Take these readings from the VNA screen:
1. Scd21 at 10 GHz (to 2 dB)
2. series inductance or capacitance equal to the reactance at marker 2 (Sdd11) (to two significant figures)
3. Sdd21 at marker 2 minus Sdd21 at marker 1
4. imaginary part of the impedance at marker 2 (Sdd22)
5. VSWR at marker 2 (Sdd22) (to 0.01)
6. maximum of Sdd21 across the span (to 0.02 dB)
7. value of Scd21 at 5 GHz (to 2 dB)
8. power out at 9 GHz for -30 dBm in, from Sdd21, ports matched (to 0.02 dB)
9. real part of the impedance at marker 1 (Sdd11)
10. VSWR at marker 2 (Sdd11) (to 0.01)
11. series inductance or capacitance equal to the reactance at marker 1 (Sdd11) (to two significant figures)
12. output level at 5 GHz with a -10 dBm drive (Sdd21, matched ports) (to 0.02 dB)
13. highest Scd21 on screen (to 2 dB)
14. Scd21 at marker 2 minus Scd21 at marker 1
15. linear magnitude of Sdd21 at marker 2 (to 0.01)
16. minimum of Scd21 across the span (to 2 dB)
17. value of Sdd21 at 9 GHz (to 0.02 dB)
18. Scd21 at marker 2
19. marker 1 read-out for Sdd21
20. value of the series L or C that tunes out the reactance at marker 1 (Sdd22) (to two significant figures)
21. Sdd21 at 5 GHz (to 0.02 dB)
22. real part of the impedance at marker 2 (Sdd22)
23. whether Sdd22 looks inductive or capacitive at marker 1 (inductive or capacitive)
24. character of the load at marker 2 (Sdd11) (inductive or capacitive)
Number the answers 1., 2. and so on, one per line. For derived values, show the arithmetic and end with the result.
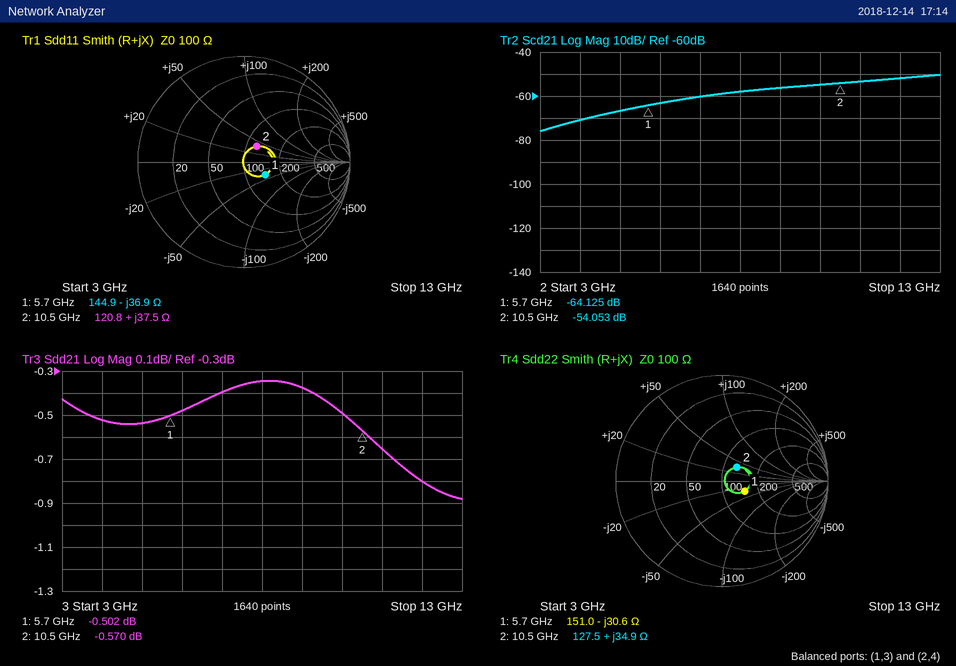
1. -54 dB
2. L = 37.5 Ω/(2π × 10.5 GHz) ≈ 568 pH, so 570 pH to two significant figures
3. -0.57 − (-0.502) = -0.068 dB
4. +34.9 Ω
5. 1.48
6. -0.34 dB
7. -66 dB
8. -30 dBm + (-0.38 dB) = -30.38 dBm
9. 144.9 Ω
10. 1.47
11. C = 1/(2π × 5.7 GHz × 36.9 Ω) ≈ 757 fF, so 760 fF to two significant figures
12. -10 dBm + (-0.54 dB) = -10.54 dBm
13. -50 dB
14. -54.053 − (-64.125) = 10.072 dB
15. 10^(-0.57/20) ≈ 0.94
16. -76 dB
17. -0.38 dB
18. -54.053 dB
19. -0.502 dB
20. L = 30.6 Ω/(2π × 5.7 GHz) ≈ 854 pH, so 850 pH to two significant figures
21. -0.54 dB
22. 127.5 Ω
23. capacitive
24. inductive
